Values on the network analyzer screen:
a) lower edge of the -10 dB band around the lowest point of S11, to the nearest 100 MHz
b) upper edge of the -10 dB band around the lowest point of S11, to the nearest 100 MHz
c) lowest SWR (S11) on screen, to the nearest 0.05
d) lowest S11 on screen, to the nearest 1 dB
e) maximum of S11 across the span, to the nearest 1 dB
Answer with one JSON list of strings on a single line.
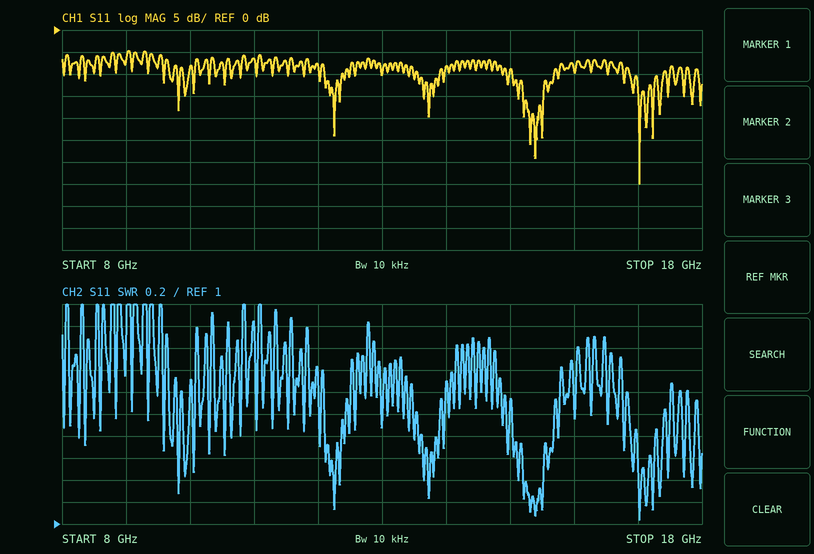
["16.9 GHz", "17.4 GHz", "1.05", "-35 dB", "-5 dB"]
